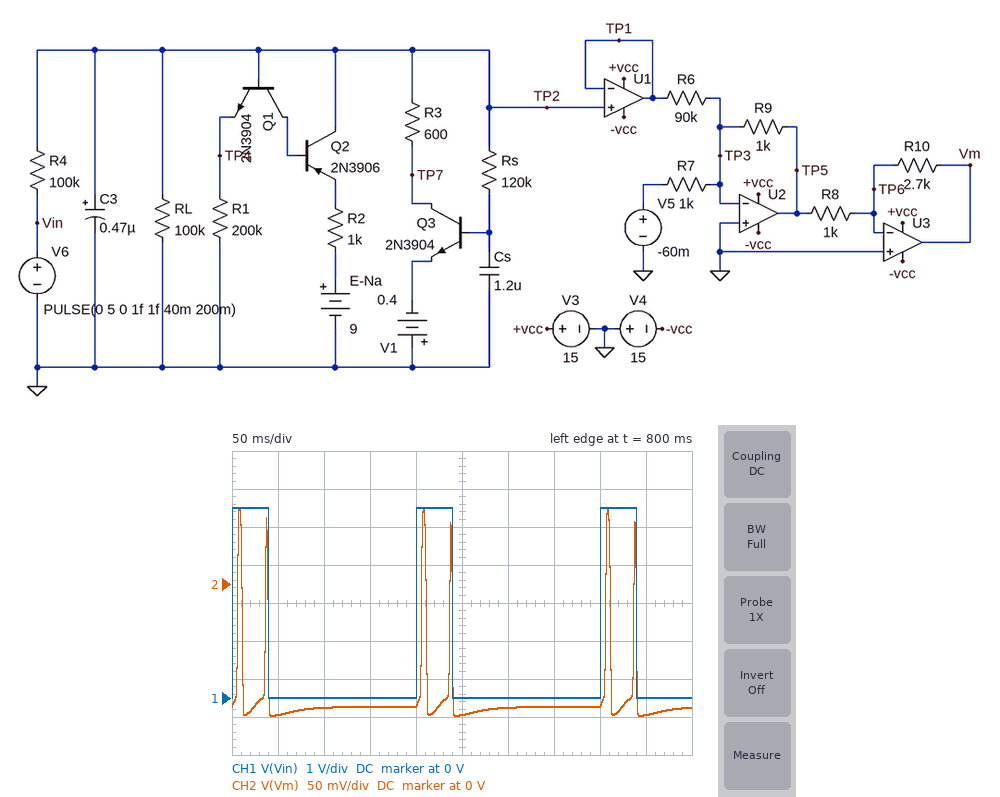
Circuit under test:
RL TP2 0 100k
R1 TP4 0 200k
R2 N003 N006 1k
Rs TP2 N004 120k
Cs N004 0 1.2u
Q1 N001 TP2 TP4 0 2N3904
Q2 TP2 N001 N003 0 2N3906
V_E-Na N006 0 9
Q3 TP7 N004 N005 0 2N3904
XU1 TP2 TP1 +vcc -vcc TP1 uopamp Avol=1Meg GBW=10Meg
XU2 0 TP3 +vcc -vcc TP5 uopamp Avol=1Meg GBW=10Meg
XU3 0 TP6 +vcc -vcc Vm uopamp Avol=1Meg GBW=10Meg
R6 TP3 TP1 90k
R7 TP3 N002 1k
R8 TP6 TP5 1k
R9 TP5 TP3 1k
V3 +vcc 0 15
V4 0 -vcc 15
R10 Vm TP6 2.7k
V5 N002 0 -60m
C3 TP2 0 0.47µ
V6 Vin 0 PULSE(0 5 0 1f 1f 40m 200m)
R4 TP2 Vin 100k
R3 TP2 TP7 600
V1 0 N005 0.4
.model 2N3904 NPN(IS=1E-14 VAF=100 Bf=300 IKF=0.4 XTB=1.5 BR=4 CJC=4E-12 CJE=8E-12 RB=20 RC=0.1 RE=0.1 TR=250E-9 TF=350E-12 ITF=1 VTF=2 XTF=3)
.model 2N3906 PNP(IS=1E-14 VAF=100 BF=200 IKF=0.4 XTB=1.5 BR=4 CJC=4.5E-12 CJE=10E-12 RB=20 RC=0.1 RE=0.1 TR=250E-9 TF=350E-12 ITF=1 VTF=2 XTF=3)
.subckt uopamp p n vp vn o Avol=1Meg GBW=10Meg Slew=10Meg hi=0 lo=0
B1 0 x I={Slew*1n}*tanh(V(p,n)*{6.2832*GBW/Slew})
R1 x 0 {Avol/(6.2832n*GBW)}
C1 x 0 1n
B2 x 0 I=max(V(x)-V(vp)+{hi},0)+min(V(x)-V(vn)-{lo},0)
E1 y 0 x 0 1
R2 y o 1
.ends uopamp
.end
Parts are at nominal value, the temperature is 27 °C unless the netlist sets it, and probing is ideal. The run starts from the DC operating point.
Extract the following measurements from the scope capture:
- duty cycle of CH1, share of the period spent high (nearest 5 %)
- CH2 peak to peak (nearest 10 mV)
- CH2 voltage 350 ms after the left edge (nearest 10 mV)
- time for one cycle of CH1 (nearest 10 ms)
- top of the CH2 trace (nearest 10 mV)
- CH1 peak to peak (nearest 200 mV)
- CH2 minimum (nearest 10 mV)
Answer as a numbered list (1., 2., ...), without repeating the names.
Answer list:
1. 20 %
2. 270 mV
3. -160 mV
4. 200 ms
5. 100 mV
6. 5.0 V
7. -170 mV
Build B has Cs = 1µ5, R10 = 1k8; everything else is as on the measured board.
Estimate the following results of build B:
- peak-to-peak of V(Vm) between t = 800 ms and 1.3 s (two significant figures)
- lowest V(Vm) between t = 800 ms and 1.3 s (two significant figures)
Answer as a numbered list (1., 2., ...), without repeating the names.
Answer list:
1. 180 mV
2. -120 mV
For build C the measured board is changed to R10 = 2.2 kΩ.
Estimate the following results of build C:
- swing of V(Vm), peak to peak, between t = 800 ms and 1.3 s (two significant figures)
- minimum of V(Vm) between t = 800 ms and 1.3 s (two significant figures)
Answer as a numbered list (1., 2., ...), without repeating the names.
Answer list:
1. 220 mV
2. -140 mV
